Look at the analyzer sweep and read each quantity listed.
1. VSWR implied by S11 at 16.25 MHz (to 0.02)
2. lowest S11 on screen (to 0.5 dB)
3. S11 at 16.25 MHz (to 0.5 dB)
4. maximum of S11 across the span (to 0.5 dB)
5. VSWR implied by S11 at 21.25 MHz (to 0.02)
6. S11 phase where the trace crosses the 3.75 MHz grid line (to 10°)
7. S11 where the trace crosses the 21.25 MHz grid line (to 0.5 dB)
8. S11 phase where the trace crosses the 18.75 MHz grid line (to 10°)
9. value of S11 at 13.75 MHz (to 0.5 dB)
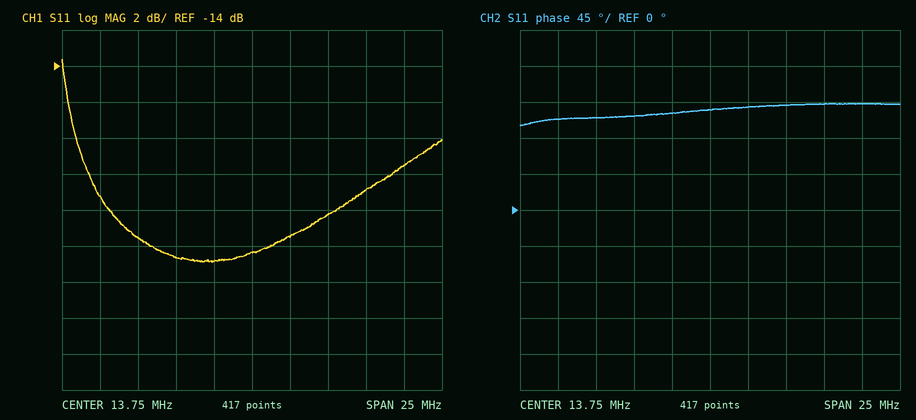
1.14
-25.0 dB
-23.5 dB
-13.5 dB
1.20
110°
-21.0 dB
130°
-24.5 dB
